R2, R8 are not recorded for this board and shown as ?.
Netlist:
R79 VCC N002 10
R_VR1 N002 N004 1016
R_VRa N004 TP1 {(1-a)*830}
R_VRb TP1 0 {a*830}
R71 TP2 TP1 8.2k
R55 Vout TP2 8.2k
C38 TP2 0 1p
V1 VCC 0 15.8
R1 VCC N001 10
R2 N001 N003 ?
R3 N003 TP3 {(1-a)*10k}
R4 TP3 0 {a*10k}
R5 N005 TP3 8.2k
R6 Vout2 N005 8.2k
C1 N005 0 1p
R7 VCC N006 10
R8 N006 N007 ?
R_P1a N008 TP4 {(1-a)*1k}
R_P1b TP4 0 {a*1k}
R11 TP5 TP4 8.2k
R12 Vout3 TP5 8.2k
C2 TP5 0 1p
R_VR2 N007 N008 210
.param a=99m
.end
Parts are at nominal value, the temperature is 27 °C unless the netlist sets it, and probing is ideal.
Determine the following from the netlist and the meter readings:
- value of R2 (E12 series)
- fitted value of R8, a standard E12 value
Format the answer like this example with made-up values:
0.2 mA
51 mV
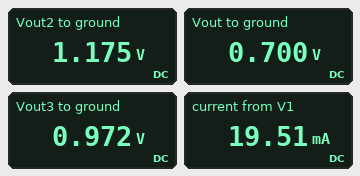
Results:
3.3 kΩ
390 Ω
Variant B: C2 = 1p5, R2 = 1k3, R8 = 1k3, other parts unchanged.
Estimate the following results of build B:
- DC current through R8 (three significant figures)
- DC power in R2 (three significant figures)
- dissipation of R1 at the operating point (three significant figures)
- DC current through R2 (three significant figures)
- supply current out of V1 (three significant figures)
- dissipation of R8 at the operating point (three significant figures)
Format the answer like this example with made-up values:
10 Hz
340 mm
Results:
6.27 mA
2.54 mW
19.5 µW
1.40 mA
16.2 mA
51.1 mW
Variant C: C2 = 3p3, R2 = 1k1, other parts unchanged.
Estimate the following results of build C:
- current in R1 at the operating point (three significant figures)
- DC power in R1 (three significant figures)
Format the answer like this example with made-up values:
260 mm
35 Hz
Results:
1.42 mA
20.2 µW
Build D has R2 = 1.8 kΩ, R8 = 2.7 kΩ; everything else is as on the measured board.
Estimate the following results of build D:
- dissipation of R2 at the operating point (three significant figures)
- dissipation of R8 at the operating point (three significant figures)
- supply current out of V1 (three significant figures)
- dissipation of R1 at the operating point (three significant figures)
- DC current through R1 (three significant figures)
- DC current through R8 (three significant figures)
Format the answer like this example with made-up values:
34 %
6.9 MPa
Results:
3.22 mW
43.9 mW
13.9 mA
17.9 µW
1.34 mA
4.03 mA
